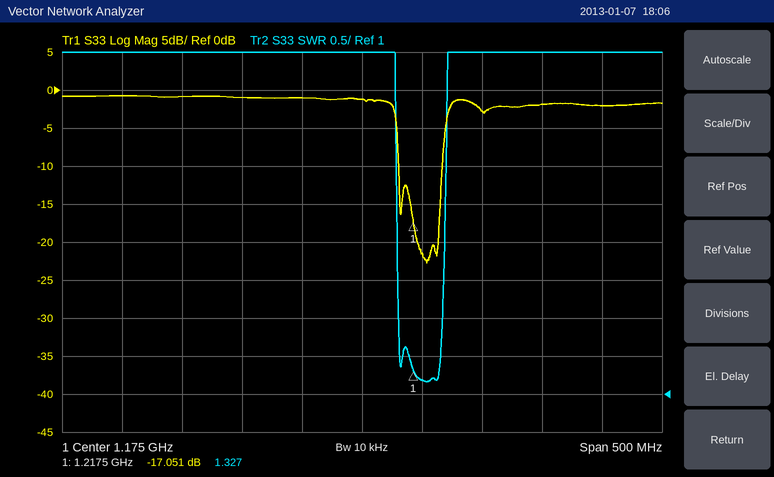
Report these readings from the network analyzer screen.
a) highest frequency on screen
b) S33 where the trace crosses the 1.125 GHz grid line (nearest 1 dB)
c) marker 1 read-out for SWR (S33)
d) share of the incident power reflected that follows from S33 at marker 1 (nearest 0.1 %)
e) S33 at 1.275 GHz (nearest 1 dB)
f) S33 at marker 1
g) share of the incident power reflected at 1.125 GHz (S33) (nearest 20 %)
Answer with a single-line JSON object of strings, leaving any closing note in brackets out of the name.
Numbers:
{"highest frequency on screen": "1.425 GHz", "S33 where the trace crosses the 1.125 GHz grid line": "-1 dB", "marker 1 read-out for SWR": "1.327", "share of the incident power reflected that follows from S33 at marker 1": "2.0 %", "S33 at 1.275 GHz": "-3 dB", "S33 at marker 1": "-17.051 dB", "share of the incident power reflected at 1.125 GHz (S33)": "80 %"}
